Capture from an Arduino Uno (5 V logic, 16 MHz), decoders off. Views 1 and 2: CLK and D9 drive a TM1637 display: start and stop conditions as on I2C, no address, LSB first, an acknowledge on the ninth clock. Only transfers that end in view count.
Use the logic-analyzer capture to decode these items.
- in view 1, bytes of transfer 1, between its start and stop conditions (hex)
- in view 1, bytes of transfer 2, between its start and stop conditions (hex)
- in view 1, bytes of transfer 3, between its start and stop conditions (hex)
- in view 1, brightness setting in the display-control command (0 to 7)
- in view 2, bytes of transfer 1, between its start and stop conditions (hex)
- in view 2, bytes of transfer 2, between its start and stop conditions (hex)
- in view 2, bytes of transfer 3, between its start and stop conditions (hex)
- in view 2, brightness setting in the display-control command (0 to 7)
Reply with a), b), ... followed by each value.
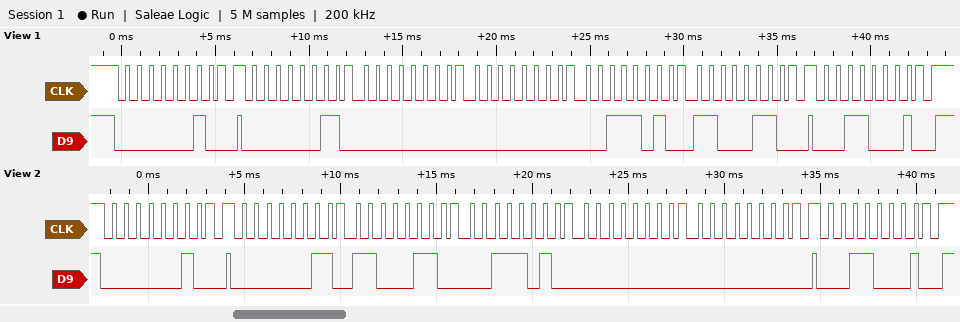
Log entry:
a) 40
b) C0 00 00 5C 63
c) 8C
d) 4
e) 40
f) C0 63 5C 00 00
g) 8C
h) 4
